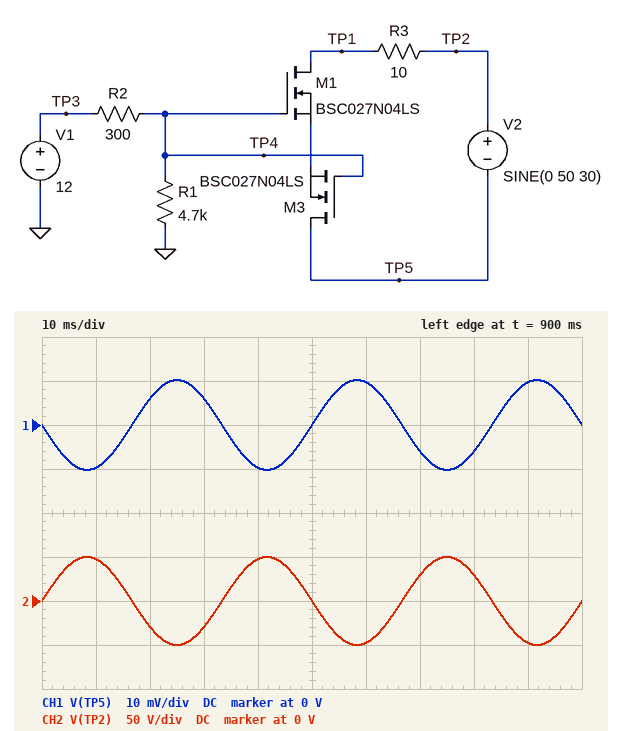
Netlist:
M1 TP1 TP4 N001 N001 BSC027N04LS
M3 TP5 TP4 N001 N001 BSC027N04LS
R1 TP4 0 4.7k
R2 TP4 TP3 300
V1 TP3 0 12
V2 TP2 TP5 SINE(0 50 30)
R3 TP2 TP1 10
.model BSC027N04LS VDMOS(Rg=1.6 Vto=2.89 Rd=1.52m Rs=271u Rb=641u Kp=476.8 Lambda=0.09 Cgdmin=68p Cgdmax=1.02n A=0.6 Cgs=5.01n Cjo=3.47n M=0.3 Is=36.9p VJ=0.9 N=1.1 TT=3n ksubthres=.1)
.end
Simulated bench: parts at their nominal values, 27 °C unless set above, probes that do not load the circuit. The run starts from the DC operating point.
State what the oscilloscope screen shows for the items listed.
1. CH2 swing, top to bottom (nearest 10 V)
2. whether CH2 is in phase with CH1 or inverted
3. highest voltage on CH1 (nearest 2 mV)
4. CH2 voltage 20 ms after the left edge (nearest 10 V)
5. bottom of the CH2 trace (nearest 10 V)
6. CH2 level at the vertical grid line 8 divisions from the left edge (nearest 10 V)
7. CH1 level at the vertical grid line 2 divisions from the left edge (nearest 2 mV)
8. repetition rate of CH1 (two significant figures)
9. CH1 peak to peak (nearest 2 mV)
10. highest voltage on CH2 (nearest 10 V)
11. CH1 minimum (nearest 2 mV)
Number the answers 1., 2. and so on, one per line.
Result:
1. 100 V
2. inverted
3. 10 mV
4. -30 V
5. -50 V
6. 30 V
7. 6 mV
8. 30 Hz
9. 20 mV
10. 50 V
11. -10 mV
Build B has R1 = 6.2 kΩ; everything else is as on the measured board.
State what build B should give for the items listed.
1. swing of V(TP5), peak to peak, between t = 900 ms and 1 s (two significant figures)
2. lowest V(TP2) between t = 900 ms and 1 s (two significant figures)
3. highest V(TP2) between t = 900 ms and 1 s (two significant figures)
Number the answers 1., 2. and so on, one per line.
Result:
1. 50 V
2. 10 V
3. 60 V
